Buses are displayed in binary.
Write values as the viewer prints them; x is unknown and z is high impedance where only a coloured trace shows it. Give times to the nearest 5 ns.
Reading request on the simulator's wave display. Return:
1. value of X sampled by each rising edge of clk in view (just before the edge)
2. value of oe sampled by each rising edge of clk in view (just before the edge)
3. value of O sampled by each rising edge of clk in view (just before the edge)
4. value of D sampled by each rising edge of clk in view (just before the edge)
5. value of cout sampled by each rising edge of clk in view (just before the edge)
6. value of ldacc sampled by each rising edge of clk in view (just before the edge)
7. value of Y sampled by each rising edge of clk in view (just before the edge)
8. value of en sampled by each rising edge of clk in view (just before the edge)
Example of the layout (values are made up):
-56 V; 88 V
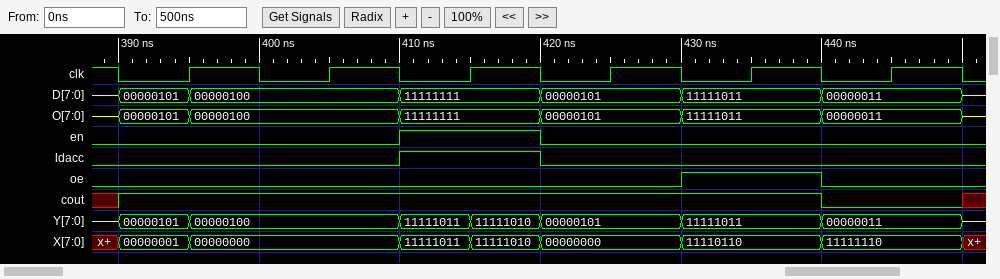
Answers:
00000001, 00000000, 11111011, 00000000, 11110110, 11111110; 0 0 0 0 1 0; 00000101, 00000100, 11111111, 00000101, 11111011, 00000011; 00000101, 00000100, 11111111, 00000101, 11111011, 00000011; 1 1 1 1 1 0; 0 0 1 0 0 0; 00000101, 00000100, 11111011, 00000101, 11111011, 00000011; 0 0 1 0 0 0
